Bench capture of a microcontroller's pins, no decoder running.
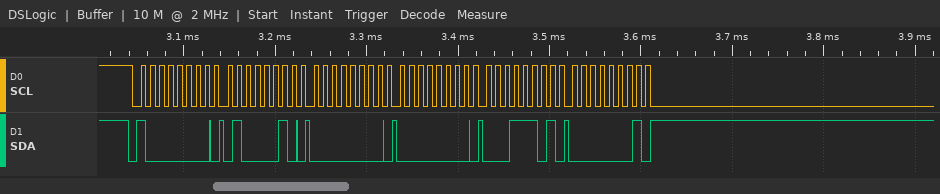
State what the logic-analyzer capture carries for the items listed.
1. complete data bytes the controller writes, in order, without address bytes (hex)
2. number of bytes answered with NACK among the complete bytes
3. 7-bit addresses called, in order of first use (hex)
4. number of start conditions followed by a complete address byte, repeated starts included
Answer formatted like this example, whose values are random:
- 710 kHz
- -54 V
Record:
- 42 00 00 1D 01
- 0
- 0x40
- 1
